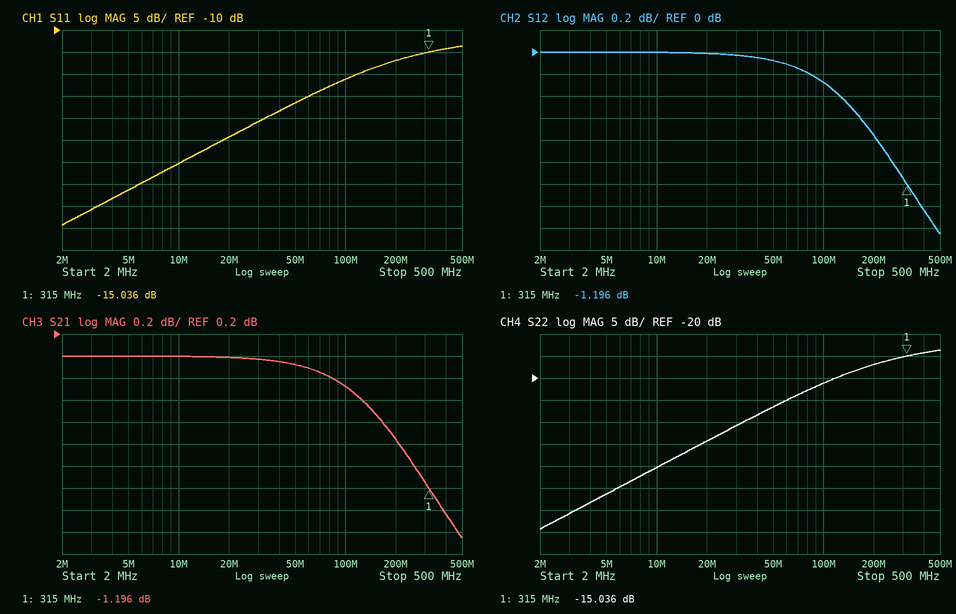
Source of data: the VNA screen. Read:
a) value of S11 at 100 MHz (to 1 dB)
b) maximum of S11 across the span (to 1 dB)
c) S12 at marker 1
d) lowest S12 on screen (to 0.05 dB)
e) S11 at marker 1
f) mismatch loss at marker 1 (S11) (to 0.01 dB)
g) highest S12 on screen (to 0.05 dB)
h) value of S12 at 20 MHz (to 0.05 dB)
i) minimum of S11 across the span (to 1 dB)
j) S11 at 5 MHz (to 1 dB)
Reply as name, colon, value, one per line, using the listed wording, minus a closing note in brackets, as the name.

value of S11 at 100 MHz: -21 dB
maximum of S11 across the span: -14 dB
S12 at marker 1: -1.196 dB
lowest S12 on screen: -1.65 dB
S11 at marker 1: -15.036 dB
mismatch loss at marker 1 (S11): 0.14 dB
highest S12 on screen: 0.00 dB
value of S12 at 20 MHz: 0.00 dB
minimum of S11 across the span: -54 dB
S11 at 5 MHz: -46 dB
